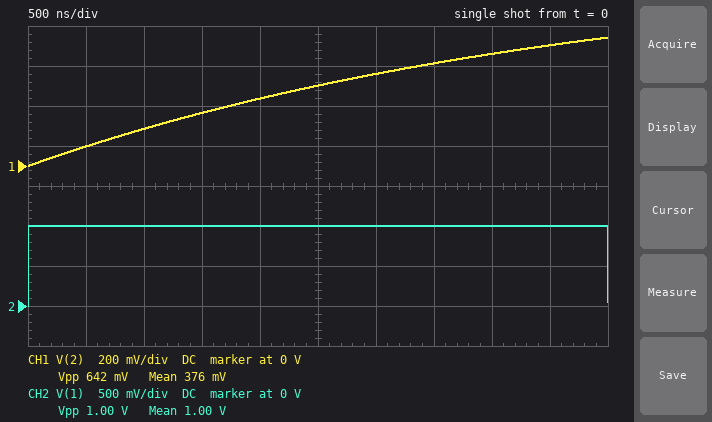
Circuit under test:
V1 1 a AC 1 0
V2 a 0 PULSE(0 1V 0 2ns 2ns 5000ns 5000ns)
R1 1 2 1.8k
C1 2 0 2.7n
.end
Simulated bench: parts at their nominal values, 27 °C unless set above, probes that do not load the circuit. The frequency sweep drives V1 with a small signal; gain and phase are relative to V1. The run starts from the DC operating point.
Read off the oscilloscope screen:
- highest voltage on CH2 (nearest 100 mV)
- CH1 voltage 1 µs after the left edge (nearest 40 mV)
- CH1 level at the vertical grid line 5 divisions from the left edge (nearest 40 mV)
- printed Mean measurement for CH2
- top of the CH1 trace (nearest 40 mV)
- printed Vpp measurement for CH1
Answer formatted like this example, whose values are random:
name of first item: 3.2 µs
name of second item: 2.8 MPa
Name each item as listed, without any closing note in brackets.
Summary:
highest voltage on CH2: 1.0 V
CH1 voltage 1 µs after the left edge: 200 mV
CH1 level at the vertical grid line 5 divisions from the left edge: 400 mV
printed Mean measurement for CH2: 1.00 V
top of the CH1 trace: 640 mV
printed Vpp measurement for CH1: 642 mV
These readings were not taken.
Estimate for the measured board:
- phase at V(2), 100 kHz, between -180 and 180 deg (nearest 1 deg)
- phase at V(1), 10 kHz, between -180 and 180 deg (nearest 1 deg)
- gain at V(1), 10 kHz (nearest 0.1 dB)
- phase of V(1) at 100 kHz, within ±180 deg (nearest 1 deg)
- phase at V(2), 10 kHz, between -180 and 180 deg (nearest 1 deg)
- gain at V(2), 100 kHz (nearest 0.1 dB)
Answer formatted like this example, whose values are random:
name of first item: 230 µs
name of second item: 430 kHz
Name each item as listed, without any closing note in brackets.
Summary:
phase at V(2), 100 kHz, between -180 and 180 deg: -72 deg
phase at V(1), 10 kHz, between -180 and 180 deg: 0 deg
gain at V(1), 10 kHz: 0 dB
phase of V(1) at 100 kHz, within ±180 deg: 0 deg
phase at V(2), 10 kHz, between -180 and 180 deg: -17 deg
gain at V(2), 100 kHz: -10.1 dB
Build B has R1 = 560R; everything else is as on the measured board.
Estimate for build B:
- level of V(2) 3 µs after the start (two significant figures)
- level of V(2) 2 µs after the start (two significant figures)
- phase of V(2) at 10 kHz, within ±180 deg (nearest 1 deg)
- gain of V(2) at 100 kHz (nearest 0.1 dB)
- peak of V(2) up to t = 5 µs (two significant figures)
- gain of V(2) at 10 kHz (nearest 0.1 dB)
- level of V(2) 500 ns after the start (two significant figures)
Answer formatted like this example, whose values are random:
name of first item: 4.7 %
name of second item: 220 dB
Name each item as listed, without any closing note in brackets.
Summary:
level of V(2) 3 µs after the start: 860 mV
level of V(2) 2 µs after the start: 730 mV
phase of V(2) at 10 kHz, within ±180 deg: -5 deg
gain of V(2) at 100 kHz: -2.8 dB
peak of V(2) up to t = 5 µs: 960 mV
gain of V(2) at 10 kHz: 0 dB
level of V(2) 500 ns after the start: 280 mV
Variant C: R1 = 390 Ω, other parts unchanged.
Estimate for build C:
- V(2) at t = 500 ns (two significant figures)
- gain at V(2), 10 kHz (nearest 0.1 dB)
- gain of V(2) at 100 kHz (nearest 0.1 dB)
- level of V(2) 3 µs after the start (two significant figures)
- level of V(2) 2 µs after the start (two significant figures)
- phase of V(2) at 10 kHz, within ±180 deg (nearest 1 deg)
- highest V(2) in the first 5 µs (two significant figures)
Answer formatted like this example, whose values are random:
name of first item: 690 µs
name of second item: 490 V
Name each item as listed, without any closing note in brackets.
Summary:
V(2) at t = 500 ns: 380 mV
gain at V(2), 10 kHz: 0 dB
gain of V(2) at 100 kHz: -1.6 dB
level of V(2) 3 µs after the start: 940 mV
level of V(2) 2 µs after the start: 850 mV
phase of V(2) at 10 kHz, within ±180 deg: -4 deg
highest V(2) in the first 5 µs: 990 mV
